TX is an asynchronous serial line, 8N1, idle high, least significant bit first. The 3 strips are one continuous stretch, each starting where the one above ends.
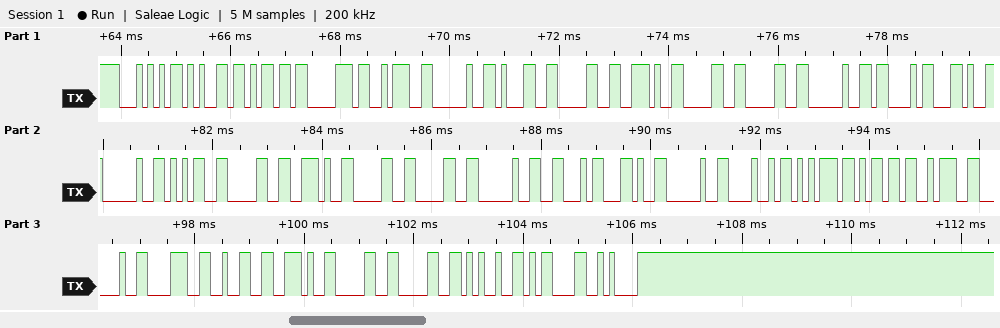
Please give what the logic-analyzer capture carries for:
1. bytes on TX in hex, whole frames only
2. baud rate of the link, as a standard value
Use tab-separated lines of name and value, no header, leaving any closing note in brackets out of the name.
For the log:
bytes on TX in hex, whole frames only	54 65 6D 70 3A 20 31 30 2E 30 30 20 43 2C 20 35 30 2E 30 30 20 46 2C 20 48 75 6D 3A 20 38 32 2E 30 30 25 0D 0A
baud rate of the link, as a standard value	9600 baud
